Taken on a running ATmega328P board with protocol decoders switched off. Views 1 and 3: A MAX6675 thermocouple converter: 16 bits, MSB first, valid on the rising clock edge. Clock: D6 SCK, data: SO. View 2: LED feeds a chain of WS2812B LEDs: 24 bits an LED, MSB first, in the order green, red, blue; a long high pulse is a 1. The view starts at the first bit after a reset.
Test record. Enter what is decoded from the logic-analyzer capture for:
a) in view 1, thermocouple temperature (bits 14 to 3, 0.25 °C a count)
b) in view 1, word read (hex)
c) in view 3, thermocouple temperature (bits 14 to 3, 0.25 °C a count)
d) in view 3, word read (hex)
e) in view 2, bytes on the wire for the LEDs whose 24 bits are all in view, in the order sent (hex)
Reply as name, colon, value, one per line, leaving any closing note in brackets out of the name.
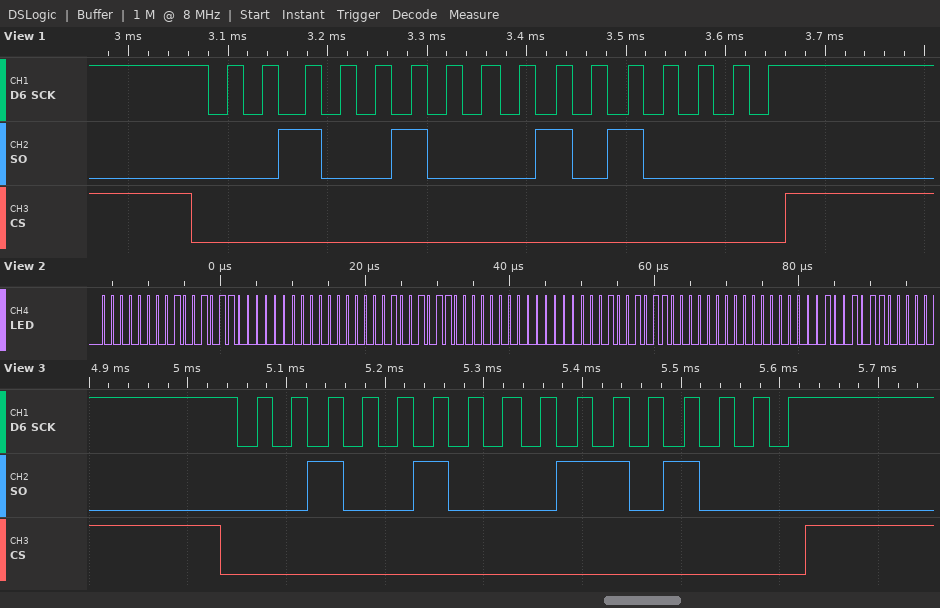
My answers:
in view 1, thermocouple temperature: 290.50 °C
in view 1, word read: 0x2450
in view 3, thermocouple temperature: 291.25 °C
in view 3, word read: 0x2468
in view 2, bytes on the wire for the LEDs whose 24 bits are all in view, in the order sent: 00 96 00 00 96 00 00 96 00
